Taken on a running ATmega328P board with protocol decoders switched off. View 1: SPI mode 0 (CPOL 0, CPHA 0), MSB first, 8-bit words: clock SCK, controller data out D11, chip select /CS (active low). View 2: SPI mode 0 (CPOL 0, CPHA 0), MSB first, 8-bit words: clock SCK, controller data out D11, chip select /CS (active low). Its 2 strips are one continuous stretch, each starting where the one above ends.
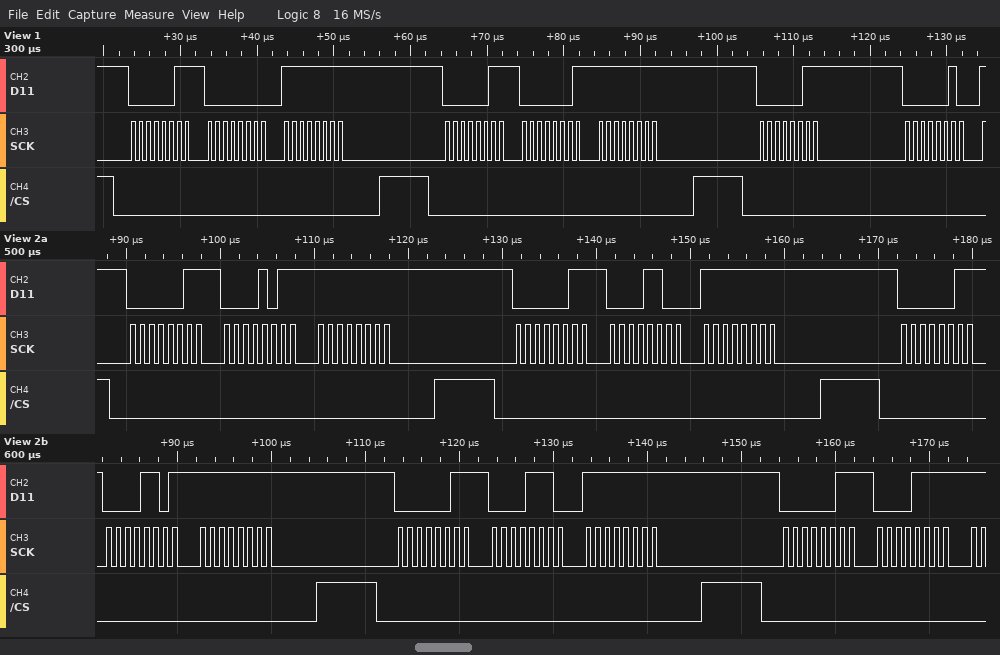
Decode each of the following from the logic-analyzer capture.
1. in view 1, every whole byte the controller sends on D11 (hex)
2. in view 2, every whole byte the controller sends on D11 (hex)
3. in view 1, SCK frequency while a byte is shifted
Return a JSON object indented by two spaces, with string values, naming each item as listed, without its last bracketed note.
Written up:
{
  "in view 1, every whole byte the controller sends on D11": "03 00 FF 03 01 FF 03 02",
  "in view 2, every whole byte the controller sends on D11": "0x03 0x0B 0xFF 0x03 0x0C 0xFF 0x03 0x0D 0xFF 0x03 0x0E 0xFF 0x03 0x0F",
  "in view 1, SCK frequency while a byte is shifted": "1 MHz"
}
